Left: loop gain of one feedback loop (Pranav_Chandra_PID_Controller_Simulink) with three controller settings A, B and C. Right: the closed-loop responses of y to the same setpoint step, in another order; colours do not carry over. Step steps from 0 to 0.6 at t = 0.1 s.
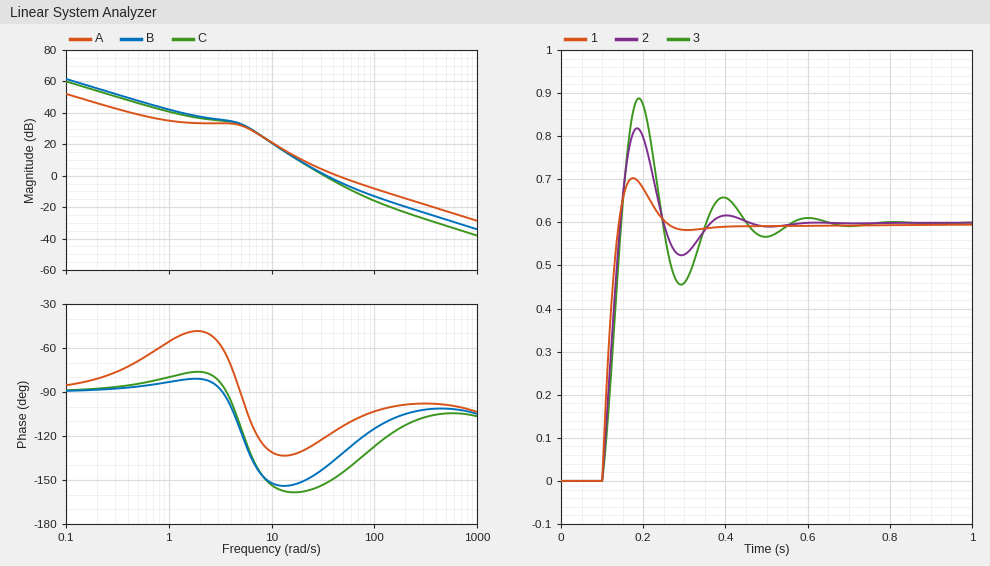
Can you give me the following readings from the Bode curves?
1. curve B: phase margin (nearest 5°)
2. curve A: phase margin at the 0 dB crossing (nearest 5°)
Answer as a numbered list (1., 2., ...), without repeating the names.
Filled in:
1. 40°
2. 65°
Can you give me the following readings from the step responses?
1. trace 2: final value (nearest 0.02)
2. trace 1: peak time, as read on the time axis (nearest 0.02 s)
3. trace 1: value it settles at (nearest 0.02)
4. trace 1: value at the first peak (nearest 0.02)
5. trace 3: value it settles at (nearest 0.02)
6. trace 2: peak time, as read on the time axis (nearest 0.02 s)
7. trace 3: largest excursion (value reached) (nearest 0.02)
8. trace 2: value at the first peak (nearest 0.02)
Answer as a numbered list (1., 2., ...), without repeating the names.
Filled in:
1. 0.60
2. 0.18 s
3. 0.60
4. 0.70
5. 0.60
6. 0.18 s
7. 0.88
8. 0.82
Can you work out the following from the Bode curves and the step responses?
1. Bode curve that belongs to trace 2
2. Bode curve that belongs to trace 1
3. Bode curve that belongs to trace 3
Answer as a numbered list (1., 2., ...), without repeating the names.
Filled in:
1. B
2. A
3. C
